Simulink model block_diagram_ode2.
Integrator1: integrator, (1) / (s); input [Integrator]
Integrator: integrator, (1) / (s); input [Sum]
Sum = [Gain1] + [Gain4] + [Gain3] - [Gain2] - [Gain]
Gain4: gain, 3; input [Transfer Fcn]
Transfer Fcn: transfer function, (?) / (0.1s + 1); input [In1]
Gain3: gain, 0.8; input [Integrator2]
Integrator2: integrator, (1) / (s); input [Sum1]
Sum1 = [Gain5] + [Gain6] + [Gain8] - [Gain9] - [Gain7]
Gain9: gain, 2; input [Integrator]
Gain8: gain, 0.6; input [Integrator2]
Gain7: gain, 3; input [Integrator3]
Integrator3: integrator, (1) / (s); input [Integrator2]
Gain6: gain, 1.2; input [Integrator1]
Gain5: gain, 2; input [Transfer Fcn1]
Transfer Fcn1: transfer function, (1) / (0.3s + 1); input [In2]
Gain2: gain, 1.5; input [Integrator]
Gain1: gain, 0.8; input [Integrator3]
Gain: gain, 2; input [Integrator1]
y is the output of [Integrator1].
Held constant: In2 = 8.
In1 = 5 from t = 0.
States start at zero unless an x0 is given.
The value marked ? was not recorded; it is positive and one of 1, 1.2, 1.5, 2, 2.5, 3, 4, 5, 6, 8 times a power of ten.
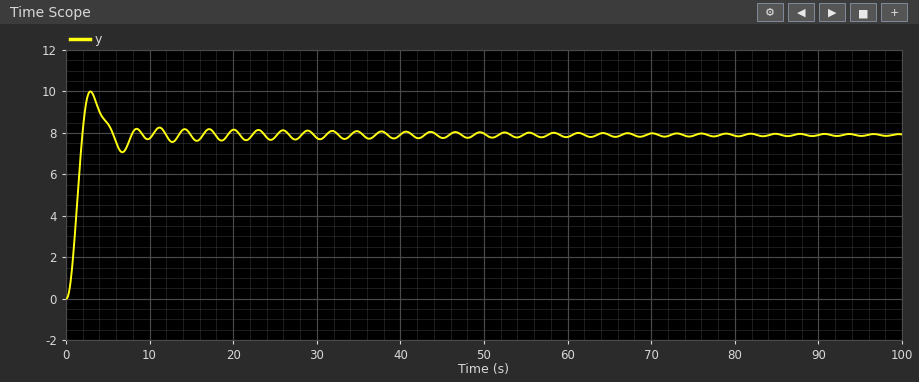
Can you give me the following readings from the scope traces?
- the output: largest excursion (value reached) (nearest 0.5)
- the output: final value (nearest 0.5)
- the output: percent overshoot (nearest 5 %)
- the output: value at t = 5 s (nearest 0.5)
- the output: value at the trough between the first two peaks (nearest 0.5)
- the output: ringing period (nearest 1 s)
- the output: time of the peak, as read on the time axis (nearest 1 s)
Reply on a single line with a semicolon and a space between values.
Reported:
10.0; 8.0; 25 %; 8.5; 7.0; 8 s; 3 s
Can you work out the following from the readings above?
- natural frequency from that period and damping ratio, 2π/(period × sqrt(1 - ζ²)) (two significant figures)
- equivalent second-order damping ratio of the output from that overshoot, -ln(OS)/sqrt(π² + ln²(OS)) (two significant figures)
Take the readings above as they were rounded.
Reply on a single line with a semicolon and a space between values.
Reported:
0.86 rad/s; 0.40
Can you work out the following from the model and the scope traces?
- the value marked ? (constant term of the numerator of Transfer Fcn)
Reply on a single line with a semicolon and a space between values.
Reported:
0.6
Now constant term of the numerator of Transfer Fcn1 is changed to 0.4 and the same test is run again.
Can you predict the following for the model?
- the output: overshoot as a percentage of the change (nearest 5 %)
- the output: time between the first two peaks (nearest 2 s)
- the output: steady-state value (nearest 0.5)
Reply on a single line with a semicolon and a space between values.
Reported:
30 %; 6 s; 6.5
